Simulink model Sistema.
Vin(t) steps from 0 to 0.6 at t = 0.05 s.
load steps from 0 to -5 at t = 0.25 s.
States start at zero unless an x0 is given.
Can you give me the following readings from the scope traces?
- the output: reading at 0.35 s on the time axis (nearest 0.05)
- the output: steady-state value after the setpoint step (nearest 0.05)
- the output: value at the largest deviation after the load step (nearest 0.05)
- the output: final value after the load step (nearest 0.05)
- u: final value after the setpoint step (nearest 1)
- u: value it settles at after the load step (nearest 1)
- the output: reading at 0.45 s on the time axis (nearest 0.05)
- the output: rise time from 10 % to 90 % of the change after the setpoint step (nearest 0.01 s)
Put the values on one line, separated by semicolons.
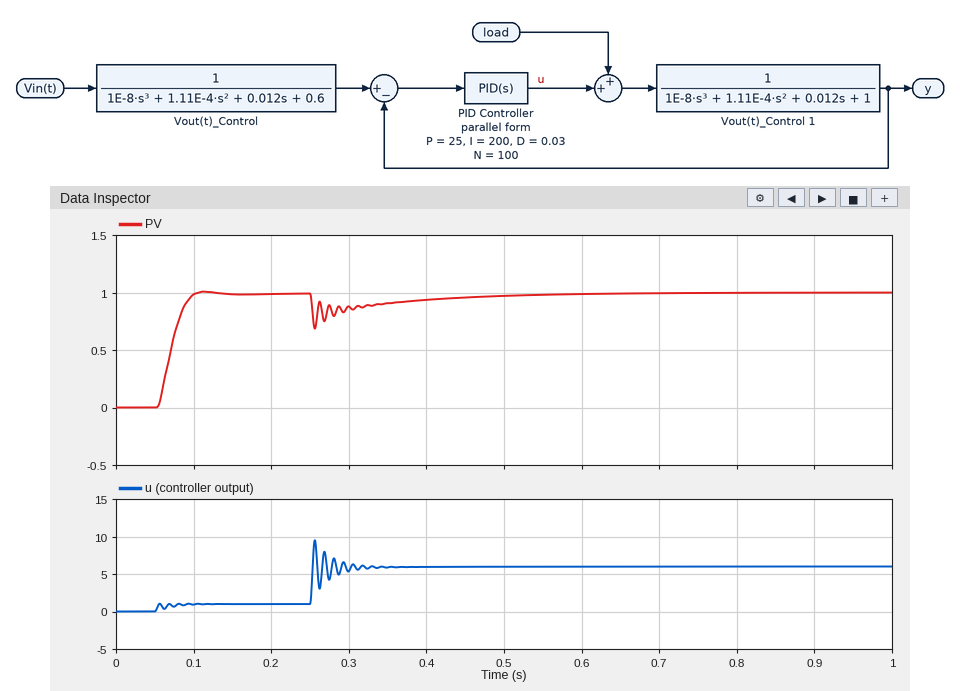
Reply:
0.90; 1.00; 0.70; 1.00; 1; 6; 0.95; 0.03 s
